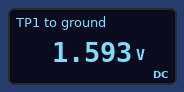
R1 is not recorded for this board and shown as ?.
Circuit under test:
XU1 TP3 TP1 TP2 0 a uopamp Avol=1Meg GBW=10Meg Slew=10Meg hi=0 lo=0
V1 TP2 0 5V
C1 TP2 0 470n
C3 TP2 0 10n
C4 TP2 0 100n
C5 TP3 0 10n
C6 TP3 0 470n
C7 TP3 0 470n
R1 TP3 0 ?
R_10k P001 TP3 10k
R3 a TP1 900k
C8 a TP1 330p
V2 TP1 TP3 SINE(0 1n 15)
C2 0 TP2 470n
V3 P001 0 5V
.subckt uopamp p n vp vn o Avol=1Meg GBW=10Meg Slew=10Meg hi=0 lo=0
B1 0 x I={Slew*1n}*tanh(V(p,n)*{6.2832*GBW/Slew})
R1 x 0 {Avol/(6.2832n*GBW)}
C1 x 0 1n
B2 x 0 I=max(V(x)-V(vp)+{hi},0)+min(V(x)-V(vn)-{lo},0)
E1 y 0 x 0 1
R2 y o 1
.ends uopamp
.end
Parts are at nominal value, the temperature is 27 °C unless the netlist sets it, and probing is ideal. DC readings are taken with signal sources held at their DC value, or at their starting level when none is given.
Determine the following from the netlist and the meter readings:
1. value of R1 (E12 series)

4.7 kΩ
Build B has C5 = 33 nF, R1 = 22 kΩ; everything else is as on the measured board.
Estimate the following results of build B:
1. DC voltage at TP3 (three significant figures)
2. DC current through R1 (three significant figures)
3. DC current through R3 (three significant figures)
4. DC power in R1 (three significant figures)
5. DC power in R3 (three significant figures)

3.41 V
155 µA
3.79 µA
529 µW
12.9 µW
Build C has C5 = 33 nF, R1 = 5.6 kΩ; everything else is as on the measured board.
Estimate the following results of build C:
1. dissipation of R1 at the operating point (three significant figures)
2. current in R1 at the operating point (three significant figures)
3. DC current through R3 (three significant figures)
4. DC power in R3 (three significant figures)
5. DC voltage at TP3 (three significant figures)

571 µW
319 µA
1.99 µA
3.55 µW
1.79 V
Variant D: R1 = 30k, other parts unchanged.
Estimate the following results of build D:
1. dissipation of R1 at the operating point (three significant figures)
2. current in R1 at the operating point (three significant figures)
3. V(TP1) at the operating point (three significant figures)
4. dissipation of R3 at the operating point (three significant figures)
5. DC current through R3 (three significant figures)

461 µW
124 µA
3.72 V
15.4 µW
4.13 µA
